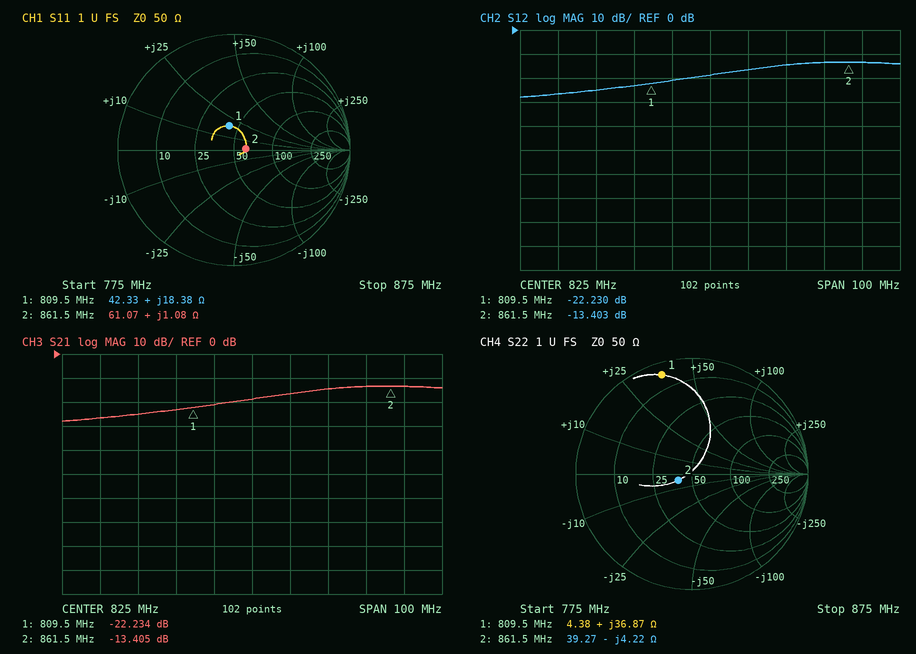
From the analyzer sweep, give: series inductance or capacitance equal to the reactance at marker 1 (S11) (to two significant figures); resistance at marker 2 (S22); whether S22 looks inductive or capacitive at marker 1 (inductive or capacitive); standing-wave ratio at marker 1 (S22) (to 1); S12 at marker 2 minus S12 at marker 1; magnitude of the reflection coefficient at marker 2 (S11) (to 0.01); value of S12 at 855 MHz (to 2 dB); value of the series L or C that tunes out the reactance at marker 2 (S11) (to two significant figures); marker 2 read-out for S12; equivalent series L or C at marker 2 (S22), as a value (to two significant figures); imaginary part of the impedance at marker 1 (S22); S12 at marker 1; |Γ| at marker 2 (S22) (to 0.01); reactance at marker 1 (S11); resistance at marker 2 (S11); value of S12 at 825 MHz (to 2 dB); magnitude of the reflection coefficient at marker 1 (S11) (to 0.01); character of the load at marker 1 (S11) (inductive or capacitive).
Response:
3.6 nH
39.27 Ω
inductive
18
8.827 dB
0.10
-14 dB
170 pF
-13.403 dB
44 pF
+36.87 Ω
-22.230 dB
0.13
+18.38 Ω
61.07 Ω
-18 dB
0.21
inductive
